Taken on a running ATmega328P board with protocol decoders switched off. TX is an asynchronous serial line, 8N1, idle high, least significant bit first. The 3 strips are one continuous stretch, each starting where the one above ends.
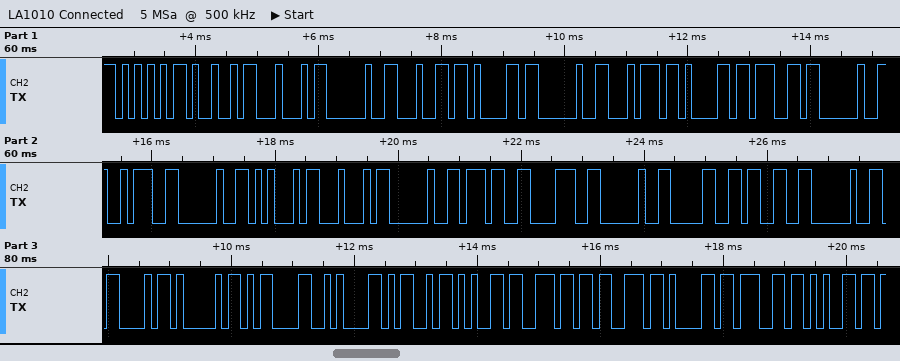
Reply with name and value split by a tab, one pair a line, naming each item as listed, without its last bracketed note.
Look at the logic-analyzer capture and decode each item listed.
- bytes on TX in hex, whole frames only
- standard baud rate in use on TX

bytes on TX in hex, whole frames only	55 49 44 20 64 61 20 74 61 67 20 3A 20 45 44 20 37 38 20 30 33 20 43 41 0D 0A 4D 65 6E 73 61 67 65
standard baud rate in use on TX	9600 baud
